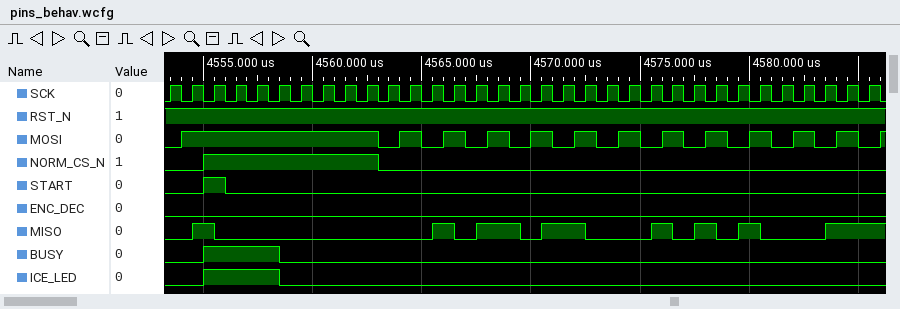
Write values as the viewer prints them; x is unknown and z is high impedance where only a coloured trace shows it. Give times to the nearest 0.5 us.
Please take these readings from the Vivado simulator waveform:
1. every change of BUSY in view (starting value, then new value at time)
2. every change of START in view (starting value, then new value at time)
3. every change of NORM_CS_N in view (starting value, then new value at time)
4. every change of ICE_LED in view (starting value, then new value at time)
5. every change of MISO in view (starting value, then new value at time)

0, 1 at 4555 us, 0 at 4558.5 us
0, 1 at 4555 us, 0 at 4556 us
0, 1 at 4555 us, 0 at 4563 us
0, 1 at 4555 us, 0 at 4558.5 us
0, 1 at 4554.5 us, 0 at 4555.5 us, 1 at 4565.5 us, 0 at 4566.5 us, 1 at 4567.5 us, 0 at 4569.5 us, 1 at 4570.5 us, 0 at 4572.5 us, 1 at 4575.5 us, 0 at 4576.5 us, 1 at 4577.5 us, 0 at 4578.5 us, 1 at 4579.5 us, 0 at 4580.5 us, 1 at 4583.5 us
